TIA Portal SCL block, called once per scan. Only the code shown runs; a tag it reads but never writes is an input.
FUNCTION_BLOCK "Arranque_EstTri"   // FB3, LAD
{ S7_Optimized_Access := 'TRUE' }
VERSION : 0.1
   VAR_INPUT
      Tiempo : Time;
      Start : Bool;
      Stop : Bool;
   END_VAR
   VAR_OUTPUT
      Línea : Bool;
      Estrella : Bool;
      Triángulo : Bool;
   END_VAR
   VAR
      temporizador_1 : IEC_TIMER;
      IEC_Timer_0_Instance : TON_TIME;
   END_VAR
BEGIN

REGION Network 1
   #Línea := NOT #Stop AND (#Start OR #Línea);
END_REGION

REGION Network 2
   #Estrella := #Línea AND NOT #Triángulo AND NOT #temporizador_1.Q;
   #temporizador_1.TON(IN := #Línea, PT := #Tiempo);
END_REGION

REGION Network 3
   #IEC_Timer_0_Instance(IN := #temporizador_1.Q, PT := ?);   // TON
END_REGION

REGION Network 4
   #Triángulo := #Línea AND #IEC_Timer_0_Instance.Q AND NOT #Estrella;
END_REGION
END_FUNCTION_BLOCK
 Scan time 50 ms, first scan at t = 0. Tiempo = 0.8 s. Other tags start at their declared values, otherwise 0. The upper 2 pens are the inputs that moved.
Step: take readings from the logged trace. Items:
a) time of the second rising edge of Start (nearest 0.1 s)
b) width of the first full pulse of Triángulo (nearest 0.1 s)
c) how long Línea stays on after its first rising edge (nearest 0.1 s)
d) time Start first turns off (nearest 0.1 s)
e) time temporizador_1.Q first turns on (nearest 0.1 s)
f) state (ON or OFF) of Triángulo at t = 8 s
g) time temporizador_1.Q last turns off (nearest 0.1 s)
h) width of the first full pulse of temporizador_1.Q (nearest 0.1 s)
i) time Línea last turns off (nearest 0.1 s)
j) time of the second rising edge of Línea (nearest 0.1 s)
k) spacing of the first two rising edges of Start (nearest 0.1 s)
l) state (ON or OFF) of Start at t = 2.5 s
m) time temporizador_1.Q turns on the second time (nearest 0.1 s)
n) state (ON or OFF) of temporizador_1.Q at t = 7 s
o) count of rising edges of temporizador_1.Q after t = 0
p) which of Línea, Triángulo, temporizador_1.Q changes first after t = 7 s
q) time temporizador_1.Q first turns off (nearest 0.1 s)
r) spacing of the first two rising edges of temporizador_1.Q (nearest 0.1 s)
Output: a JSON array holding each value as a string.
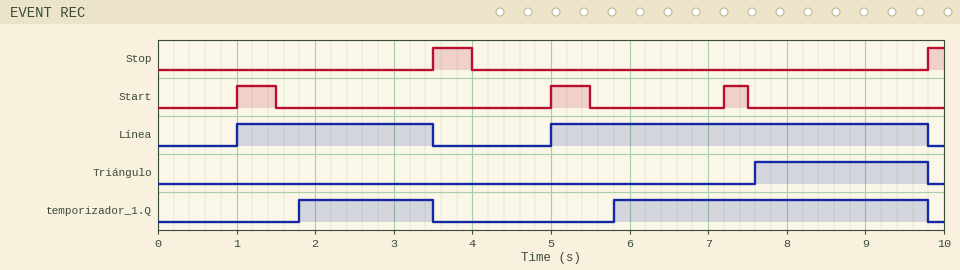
["5.0 s", "2.2 s", "2.5 s", "1.5 s", "1.8 s", "ON", "9.8 s", "1.7 s", "9.8 s", "5.0 s", "4.0 s", "OFF", "5.8 s", "ON", "2", "Triángulo", "3.5 s", "4.0 s"]
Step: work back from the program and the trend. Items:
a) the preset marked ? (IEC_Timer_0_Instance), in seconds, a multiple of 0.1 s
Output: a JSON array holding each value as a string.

["1.8 s"]
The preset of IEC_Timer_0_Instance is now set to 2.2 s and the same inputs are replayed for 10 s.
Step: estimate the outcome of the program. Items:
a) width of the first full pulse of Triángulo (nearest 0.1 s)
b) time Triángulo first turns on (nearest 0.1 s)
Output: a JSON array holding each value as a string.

["1.8 s", "8.0 s"]
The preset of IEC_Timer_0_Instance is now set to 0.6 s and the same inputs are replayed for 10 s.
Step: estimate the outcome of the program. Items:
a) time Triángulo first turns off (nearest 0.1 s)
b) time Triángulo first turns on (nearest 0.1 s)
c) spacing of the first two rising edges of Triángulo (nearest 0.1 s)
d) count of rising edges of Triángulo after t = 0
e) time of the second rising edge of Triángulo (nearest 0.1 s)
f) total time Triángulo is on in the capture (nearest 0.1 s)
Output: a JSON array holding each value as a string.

["3.5 s", "2.4 s", "4.0 s", "2", "6.4 s", "4.5 s"]
